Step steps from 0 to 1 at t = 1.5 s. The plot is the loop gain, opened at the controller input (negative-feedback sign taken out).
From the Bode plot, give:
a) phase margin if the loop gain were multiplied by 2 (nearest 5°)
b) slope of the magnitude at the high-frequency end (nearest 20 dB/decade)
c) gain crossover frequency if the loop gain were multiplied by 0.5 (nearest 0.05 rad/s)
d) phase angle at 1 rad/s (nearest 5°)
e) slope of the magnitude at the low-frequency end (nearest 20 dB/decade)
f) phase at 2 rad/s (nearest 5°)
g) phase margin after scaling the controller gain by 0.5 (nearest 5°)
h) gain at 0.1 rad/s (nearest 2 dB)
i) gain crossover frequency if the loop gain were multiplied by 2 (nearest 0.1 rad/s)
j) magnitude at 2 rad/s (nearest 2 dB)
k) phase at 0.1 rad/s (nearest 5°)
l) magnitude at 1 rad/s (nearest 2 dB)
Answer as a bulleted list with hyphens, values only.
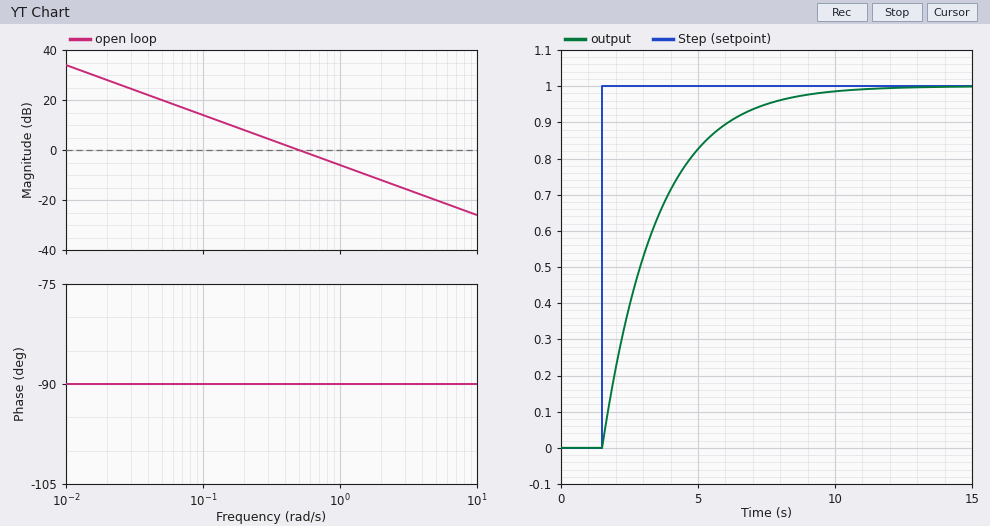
- 90°
- -20 dB/decade
- 0.25 rad/s
- -90°
- -20 dB/decade
- -90°
- 90°
- 14 dB
- 1.0 rad/s
- -12 dB
- -90°
- -6 dB
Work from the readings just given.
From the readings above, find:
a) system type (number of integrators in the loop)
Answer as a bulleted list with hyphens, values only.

- 1
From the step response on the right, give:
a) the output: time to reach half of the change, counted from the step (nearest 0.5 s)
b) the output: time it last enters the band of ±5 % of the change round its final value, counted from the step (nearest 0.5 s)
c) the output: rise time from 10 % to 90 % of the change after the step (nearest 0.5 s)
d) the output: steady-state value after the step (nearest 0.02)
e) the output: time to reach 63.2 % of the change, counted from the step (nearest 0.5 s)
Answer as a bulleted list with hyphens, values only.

- 1.5 s
- 6.0 s
- 4.5 s
- 1.00
- 2.0 s
